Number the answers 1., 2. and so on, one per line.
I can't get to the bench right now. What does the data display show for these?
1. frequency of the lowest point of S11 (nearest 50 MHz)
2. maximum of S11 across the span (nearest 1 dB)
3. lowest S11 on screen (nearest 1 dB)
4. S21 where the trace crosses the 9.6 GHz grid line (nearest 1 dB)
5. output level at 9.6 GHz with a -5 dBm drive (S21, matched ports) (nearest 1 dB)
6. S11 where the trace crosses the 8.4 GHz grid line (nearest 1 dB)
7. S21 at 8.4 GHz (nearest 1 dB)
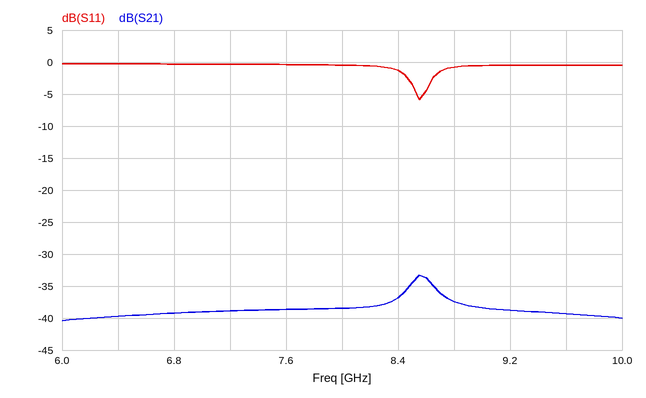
1. 8.55 GHz
2. 0 dB
3. -6 dB
4. -39 dB
5. -44 dBm
6. -1 dB
7. -37 dB
